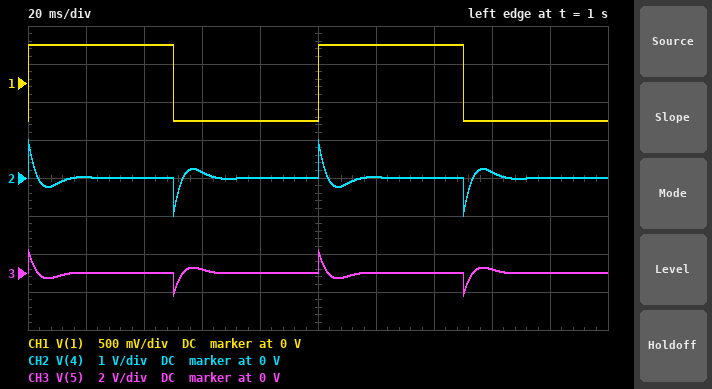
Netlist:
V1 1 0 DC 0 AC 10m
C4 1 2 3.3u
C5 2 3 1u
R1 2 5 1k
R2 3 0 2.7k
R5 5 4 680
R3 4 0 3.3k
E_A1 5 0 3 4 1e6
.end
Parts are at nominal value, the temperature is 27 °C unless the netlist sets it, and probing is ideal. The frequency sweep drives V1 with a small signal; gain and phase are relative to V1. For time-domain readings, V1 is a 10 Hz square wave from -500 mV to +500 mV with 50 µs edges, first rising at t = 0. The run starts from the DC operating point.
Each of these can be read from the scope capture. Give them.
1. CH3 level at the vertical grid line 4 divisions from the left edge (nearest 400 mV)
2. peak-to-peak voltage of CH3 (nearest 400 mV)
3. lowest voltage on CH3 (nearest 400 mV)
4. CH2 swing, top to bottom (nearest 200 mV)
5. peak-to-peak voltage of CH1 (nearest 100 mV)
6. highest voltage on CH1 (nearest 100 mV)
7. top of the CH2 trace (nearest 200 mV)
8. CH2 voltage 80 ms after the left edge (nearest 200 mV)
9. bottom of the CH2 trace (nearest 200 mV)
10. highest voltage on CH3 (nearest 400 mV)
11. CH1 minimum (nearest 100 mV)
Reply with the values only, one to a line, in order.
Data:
0 V
2.4 V
-1.2 V
2.0 V
1.0 V
500 mV
1.0 V
0 V
-1.0 V
1.2 V
-500 mV
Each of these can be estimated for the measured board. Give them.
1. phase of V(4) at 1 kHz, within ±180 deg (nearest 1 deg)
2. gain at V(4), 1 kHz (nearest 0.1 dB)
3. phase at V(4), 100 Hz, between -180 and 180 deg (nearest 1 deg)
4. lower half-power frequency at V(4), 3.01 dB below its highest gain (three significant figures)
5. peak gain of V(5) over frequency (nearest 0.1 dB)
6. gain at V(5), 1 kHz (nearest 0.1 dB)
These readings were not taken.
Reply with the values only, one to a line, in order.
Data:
4 deg
0 dB
43 deg
48.9 Hz
1.8 dB
1.6 dB
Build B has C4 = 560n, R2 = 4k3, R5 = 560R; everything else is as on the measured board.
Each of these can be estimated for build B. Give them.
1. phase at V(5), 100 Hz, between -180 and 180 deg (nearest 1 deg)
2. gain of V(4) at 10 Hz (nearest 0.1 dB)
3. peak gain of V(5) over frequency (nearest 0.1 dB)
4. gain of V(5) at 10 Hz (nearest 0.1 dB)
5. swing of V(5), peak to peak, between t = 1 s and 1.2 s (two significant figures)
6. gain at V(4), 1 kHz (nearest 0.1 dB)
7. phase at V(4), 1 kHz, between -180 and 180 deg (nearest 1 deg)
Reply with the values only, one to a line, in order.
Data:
95 deg
-40.4 dB
7.1 dB
-39.0 dB
2.3 V
0.1 dB
3 deg
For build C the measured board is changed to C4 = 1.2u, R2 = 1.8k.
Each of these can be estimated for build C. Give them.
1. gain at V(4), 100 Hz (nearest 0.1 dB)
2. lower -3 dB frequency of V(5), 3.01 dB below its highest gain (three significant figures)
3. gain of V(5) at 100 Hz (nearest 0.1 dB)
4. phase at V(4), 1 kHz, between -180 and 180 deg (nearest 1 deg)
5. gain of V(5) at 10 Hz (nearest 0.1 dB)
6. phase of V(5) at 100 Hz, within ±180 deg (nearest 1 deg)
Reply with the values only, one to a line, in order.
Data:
-2.7 dB
98.9 Hz
-1.0 dB
8 deg
-39.7 dB
97 deg
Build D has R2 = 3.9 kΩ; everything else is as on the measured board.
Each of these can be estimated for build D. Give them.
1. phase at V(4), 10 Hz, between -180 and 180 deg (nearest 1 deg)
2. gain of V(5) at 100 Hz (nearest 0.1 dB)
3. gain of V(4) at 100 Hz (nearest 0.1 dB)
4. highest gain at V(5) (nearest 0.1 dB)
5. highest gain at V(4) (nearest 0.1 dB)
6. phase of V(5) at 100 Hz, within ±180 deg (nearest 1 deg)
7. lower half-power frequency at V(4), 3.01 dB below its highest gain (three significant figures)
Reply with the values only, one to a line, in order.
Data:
167 deg
2.4 dB
0.8 dB
3.0 dB
1.4 dB
28 deg
37.8 Hz
